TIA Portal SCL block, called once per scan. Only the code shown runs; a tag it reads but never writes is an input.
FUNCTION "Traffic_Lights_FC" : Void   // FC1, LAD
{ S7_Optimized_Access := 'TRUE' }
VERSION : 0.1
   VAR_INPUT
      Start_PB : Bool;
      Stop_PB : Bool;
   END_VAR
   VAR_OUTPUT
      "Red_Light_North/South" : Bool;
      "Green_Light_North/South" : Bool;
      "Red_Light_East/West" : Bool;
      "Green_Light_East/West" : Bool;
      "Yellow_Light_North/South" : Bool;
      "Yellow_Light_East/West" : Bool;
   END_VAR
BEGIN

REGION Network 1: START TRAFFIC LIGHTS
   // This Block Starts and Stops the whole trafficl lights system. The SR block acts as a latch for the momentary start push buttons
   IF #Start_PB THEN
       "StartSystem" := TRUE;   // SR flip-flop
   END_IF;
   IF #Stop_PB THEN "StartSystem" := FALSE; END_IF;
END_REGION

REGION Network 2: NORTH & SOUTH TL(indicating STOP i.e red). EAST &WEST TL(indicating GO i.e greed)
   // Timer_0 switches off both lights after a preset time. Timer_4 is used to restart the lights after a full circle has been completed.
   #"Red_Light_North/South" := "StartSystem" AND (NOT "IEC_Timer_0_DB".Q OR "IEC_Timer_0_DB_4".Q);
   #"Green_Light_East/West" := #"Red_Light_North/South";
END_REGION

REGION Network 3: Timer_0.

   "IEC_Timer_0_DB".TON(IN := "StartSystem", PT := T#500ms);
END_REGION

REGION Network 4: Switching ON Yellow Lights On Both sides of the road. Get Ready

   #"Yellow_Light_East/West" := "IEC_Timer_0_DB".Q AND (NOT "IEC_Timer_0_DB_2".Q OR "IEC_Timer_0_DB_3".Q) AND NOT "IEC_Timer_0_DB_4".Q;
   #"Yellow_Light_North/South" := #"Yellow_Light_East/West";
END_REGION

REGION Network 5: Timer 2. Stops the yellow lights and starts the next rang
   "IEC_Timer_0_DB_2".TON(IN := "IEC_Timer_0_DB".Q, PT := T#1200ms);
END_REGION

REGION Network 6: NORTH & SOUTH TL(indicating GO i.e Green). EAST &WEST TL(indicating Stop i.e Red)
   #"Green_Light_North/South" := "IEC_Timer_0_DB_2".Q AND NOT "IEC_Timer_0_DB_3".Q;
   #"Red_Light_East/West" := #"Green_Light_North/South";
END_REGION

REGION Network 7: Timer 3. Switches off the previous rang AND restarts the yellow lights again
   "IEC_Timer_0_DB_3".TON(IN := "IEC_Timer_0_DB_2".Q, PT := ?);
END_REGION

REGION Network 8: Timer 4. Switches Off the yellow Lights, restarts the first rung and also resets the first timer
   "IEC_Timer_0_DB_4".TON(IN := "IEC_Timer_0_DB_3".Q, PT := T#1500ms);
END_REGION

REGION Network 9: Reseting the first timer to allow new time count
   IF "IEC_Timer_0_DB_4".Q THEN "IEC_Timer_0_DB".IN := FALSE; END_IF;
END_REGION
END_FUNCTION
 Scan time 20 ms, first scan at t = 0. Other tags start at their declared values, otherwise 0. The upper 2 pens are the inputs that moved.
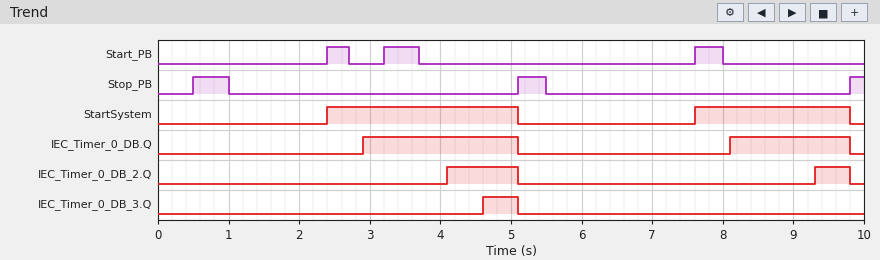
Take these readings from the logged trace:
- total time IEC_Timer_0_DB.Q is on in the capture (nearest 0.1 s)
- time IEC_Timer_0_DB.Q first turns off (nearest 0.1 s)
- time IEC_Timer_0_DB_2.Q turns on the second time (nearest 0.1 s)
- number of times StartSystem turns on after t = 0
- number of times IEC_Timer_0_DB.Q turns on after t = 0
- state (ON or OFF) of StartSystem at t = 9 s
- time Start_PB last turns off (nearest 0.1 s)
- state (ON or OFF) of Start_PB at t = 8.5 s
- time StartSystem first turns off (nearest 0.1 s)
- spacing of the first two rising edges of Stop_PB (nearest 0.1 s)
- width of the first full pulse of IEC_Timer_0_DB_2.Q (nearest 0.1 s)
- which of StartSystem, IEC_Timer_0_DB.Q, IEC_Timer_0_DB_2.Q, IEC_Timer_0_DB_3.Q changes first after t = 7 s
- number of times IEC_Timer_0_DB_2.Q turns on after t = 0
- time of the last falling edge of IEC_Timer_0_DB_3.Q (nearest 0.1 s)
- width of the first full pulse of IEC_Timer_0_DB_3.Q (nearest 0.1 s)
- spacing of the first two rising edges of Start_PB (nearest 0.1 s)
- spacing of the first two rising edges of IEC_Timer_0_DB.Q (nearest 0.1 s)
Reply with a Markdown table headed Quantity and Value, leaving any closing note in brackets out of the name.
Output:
| Quantity | Value |
|---|---|
| total time IEC_Timer_0_DB.Q is on in the capture | 3.9 s |
| time IEC_Timer_0_DB.Q first turns off | 5.1 s |
| time IEC_Timer_0_DB_2.Q turns on the second time | 9.3 s |
| number of times StartSystem turns on after t = 0 | 2 |
| number of times IEC_Timer_0_DB.Q turns on after t = 0 | 2 |
| state (ON or OFF) of StartSystem at t = 9 s | ON |
| time Start_PB last turns off | 8.0 s |
| state (ON or OFF) of Start_PB at t = 8.5 s | OFF |
| time StartSystem first turns off | 5.1 s |
| spacing of the first two rising edges of Stop_PB | 4.6 s |
| width of the first full pulse of IEC_Timer_0_DB_2.Q | 1.0 s |
| which of StartSystem, IEC_Timer_0_DB.Q, IEC_Timer_0_DB_2.Q, IEC_Timer_0_DB_3.Q changes first after t = 7 s | StartSystem |
| number of times IEC_Timer_0_DB_2.Q turns on after t = 0 | 2 |
| time of the last falling edge of IEC_Timer_0_DB_3.Q | 5.1 s |
| width of the first full pulse of IEC_Timer_0_DB_3.Q | 0.5 s |
| spacing of the first two rising edges of Start_PB | 0.8 s |
| spacing of the first two rising edges of IEC_Timer_0_DB.Q | 5.2 s |
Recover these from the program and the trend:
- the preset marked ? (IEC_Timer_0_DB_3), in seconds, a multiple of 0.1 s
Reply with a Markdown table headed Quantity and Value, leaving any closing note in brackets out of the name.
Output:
| Quantity | Value |
|---|---|
| the preset marked ? (IEC_Timer_0_DB_3), in seconds, a multiple of 0.1 s | 0.5 s |
